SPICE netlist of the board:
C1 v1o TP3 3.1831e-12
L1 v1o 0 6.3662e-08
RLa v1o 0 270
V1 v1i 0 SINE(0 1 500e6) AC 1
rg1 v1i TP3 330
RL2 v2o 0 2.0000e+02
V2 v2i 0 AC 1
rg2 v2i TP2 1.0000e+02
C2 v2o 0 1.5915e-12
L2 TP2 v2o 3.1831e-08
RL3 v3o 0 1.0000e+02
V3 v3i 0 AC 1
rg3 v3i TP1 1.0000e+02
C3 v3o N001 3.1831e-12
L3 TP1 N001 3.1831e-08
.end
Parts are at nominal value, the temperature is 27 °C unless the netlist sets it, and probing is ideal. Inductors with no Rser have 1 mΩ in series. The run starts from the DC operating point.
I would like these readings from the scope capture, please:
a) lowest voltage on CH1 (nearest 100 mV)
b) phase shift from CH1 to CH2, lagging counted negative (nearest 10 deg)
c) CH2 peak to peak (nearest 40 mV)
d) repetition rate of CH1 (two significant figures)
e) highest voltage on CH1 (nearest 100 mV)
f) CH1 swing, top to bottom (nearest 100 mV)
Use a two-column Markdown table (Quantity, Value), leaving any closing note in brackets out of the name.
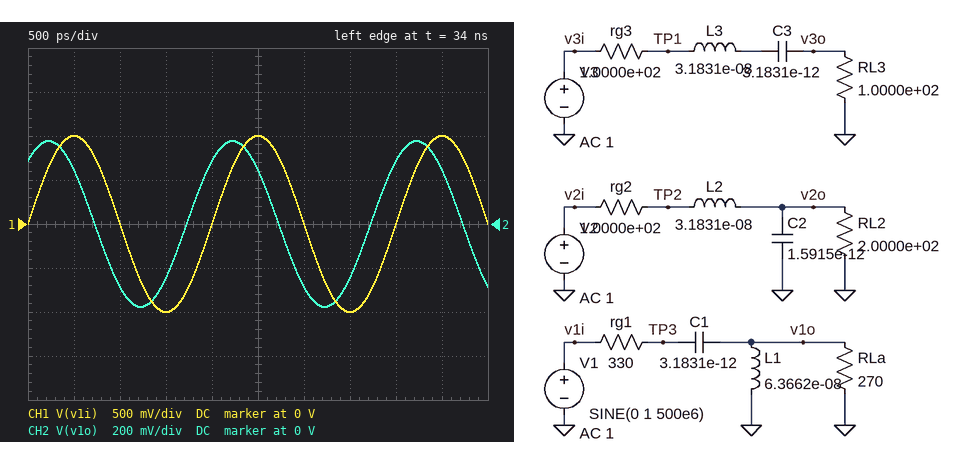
| Quantity | Value |
|---|---|
| lowest voltage on CH1 | -1.0 V |
| phase shift from CH1 to CH2, lagging counted negative | 50 deg |
| CH2 peak to peak | 760 mV |
| repetition rate of CH1 | 500 MHz |
| highest voltage on CH1 | 1.0 V |
| CH1 swing, top to bottom | 2.0 V |
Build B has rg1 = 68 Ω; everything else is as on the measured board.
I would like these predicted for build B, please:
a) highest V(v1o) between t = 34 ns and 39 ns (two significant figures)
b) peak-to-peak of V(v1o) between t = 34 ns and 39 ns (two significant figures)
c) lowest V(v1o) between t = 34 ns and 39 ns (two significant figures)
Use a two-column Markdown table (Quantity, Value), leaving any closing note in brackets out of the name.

| Quantity | Value |
|---|---|
| highest V(v1o) between t = 34 ns and 39 ns | 970 mV |
| peak-to-peak of V(v1o) between t = 34 ns and 39 ns | 1.9 V |
| lowest V(v1o) between t = 34 ns and 39 ns | -970 mV |
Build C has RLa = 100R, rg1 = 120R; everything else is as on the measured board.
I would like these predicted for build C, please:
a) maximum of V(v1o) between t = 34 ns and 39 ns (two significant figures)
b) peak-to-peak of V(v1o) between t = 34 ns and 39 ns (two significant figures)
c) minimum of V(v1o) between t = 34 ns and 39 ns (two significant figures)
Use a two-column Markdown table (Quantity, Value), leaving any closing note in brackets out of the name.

| Quantity | Value |
|---|---|
| maximum of V(v1o) between t = 34 ns and 39 ns | 430 mV |
| peak-to-peak of V(v1o) between t = 34 ns and 39 ns | 860 mV |
| minimum of V(v1o) between t = 34 ns and 39 ns | -430 mV |
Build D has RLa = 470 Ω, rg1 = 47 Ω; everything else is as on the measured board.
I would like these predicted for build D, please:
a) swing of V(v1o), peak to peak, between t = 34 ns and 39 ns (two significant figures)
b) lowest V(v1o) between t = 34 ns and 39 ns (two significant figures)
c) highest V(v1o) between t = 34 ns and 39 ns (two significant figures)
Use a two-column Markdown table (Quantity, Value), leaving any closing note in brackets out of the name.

| Quantity | Value |
|---|---|
| swing of V(v1o), peak to peak, between t = 34 ns and 39 ns | 2.7 V |
| lowest V(v1o) between t = 34 ns and 39 ns | -1.3 V |
| highest V(v1o) between t = 34 ns and 39 ns | 1.3 V |
